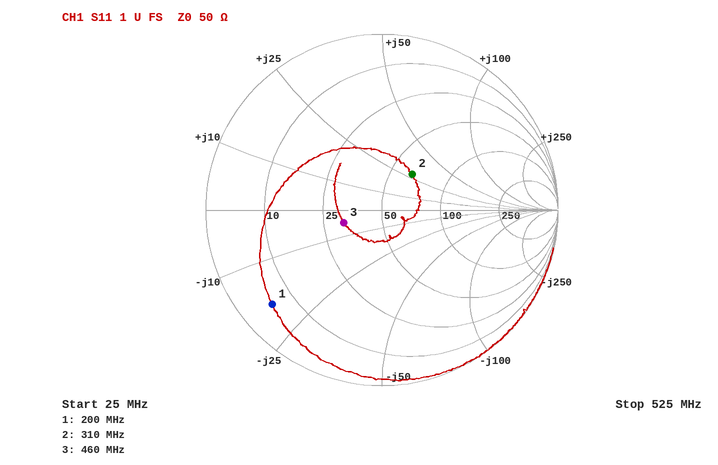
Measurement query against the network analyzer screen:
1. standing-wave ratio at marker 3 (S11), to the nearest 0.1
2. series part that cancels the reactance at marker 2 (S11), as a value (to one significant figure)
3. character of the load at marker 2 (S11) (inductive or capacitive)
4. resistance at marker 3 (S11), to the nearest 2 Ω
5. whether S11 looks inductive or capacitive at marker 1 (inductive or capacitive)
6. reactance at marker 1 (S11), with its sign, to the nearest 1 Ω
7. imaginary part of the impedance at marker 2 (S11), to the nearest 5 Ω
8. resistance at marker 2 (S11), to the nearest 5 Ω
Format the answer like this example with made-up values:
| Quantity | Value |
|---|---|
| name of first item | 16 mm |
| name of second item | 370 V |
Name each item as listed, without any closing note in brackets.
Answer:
| Quantity | Value |
|---|---|
| standing-wave ratio at marker 3 (S11), to the nearest 0.1 | 1.6 |
| series part that cancels the reactance at marker 2 (S11), as a value | 20 pF |
| character of the load at marker 2 (S11) | inductive |
| resistance at marker 3 (S11), to the nearest 2 Ω | 32 Ω |
| whether S11 looks inductive or capacitive at marker 1 | capacitive |
| reactance at marker 1 (S11), with its sign, to the nearest 1 Ω | -18 Ω |
| imaginary part of the impedance at marker 2 (S11), to the nearest 5 Ω | +30 Ω |
| resistance at marker 2 (S11), to the nearest 5 Ω | 65 Ω |
